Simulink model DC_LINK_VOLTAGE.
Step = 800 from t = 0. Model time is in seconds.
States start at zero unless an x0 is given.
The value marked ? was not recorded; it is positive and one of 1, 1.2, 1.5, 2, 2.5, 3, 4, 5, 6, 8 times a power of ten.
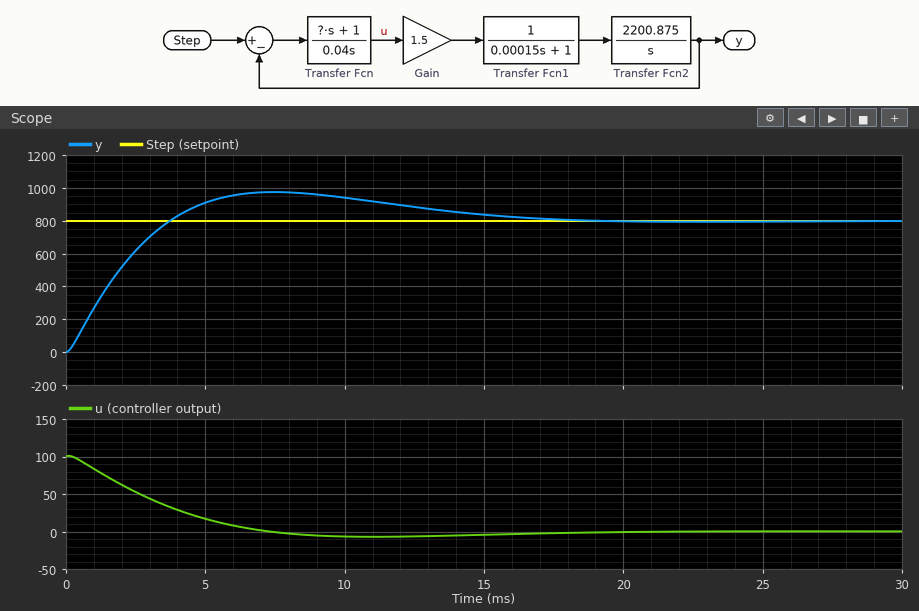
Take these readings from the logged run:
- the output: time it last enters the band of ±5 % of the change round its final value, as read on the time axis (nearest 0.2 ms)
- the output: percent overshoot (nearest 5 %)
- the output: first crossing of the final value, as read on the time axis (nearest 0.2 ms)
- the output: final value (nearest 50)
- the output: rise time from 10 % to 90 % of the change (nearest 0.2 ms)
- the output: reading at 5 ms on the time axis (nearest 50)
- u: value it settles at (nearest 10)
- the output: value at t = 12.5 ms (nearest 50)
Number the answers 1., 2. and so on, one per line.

1. 14.8 ms
2. 20 %
3. 3.8 ms
4. 800
5. 2.8 ms
6. 900
7. 0
8. 900
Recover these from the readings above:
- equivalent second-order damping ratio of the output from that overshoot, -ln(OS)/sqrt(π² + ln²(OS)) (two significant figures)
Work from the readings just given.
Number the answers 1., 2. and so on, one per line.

1. 0.46
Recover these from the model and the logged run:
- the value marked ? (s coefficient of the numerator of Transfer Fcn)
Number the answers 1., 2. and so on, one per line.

1. 0.005
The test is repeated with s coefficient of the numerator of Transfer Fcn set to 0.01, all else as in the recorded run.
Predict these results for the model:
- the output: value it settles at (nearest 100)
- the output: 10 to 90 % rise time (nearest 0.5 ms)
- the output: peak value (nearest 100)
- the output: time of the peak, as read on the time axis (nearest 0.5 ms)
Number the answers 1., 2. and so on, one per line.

1. 800
2. 2.0 ms
3. 900
4. 5.5 ms
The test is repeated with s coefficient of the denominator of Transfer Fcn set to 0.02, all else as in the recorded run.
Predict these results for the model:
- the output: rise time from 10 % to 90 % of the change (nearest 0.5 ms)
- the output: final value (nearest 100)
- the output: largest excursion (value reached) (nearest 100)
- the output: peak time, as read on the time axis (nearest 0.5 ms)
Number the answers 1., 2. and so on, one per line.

1. 1.5 ms
2. 800
3. 900
4. 4.5 ms
